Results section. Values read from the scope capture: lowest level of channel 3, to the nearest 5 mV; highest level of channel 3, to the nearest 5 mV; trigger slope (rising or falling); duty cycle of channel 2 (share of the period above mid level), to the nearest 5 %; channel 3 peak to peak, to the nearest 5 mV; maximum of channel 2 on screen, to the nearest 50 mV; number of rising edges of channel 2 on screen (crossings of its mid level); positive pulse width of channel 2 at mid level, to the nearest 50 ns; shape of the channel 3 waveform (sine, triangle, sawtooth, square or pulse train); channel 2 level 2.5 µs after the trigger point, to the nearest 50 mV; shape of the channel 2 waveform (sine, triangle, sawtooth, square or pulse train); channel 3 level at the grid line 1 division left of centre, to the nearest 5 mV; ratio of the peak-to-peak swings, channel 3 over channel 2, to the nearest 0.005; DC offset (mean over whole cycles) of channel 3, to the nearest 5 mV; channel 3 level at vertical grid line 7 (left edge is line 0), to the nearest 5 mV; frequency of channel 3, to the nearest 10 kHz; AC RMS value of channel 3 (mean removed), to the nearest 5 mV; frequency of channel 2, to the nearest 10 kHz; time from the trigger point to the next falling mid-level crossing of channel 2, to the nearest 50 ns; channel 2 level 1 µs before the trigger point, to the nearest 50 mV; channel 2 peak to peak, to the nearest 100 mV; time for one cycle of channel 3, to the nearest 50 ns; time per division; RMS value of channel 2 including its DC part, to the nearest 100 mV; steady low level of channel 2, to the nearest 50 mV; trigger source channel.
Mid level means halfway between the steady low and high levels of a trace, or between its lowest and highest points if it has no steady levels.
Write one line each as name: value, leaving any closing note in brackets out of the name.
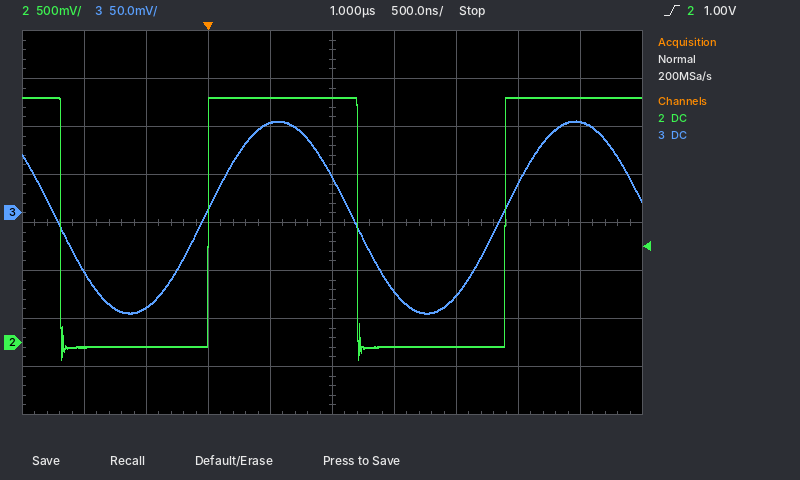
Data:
lowest level of channel 3, to the nearest 5 mV: -105 mV
highest level of channel 3, to the nearest 5 mV: 95 mV
trigger slope: rising
duty cycle of channel 2 (share of the period above mid level), to the nearest 5 %: 50 %
channel 3 peak to peak, to the nearest 5 mV: 200 mV
maximum of channel 2 on screen, to the nearest 50 mV: 2.55 V
number of rising edges of channel 2 on screen: 2
positive pulse width of channel 2 at mid level, to the nearest 50 ns: 1.20 µs
shape of the channel 3 waveform: sine
channel 2 level 2.5 µs after the trigger point, to the nearest 50 mV: 2.55 V
shape of the channel 2 waveform: square
channel 3 level at the grid line 1 division left of centre, to the nearest 5 mV: 95 mV
ratio of the peak-to-peak swings, channel 3 over channel 2, to the nearest 0.005: 0.075
DC offset (mean over whole cycles) of channel 3, to the nearest 5 mV: -5 mV
channel 3 level at vertical grid line 7 (left edge is line 0), to the nearest 5 mV: -85 mV
frequency of channel 3, to the nearest 10 kHz: 420 kHz
AC RMS value of channel 3 (mean removed), to the nearest 5 mV: 70 mV
frequency of channel 2, to the nearest 10 kHz: 420 kHz
time from the trigger point to the next falling mid-level crossing of channel 2, to the nearest 50 ns: 1.20 µs
channel 2 level 1 µs before the trigger point, to the nearest 50 mV: -50 mV
channel 2 peak to peak, to the nearest 100 mV: 2.70 V
time for one cycle of channel 3, to the nearest 50 ns: 2.40 µs
time per division: 500 ns
RMS value of channel 2 including its DC part, to the nearest 100 mV: 1.8 V
steady low level of channel 2, to the nearest 50 mV: -50 mV
trigger source channel: channel 2
